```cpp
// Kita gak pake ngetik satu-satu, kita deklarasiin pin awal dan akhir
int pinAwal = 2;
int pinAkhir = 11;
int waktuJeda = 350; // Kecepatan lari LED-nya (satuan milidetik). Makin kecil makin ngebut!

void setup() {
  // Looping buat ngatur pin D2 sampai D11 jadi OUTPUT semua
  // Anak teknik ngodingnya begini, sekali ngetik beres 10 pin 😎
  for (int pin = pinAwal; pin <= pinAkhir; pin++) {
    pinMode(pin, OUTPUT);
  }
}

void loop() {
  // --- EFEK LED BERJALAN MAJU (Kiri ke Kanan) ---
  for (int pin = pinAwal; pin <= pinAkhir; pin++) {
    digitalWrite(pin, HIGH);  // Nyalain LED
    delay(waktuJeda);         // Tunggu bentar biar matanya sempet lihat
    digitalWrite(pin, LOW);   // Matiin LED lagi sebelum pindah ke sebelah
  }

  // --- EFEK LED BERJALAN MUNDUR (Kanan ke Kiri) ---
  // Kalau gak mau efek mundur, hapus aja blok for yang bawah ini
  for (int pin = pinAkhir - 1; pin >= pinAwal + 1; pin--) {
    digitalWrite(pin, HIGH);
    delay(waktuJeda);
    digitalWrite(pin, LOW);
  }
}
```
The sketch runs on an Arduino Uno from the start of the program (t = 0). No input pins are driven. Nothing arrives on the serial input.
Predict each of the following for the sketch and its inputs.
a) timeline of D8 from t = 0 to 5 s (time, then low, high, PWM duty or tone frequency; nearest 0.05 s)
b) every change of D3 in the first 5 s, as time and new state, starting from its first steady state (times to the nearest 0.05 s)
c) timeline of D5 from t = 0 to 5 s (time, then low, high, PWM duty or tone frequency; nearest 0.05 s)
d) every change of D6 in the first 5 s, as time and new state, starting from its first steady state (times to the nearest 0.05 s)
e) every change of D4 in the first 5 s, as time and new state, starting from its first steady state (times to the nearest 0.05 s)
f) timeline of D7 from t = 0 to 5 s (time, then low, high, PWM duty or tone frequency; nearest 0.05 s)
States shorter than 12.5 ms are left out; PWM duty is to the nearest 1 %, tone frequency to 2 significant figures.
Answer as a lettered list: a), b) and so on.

a) 0 s low; 2.1 s high; 2.45 s low; 4.2 s high; 4.55 s low
b) 0 s low; 0.35 s high; 0.7 s low
c) 0 s low; 1.05 s high; 1.4 s low
d) 0 s low; 1.4 s high; 1.75 s low; 4.9 s high
e) 0 s low; 0.7 s high; 1.05 s low
f) 0 s low; 1.75 s high; 2.1 s low; 4.55 s high; 4.9 s low
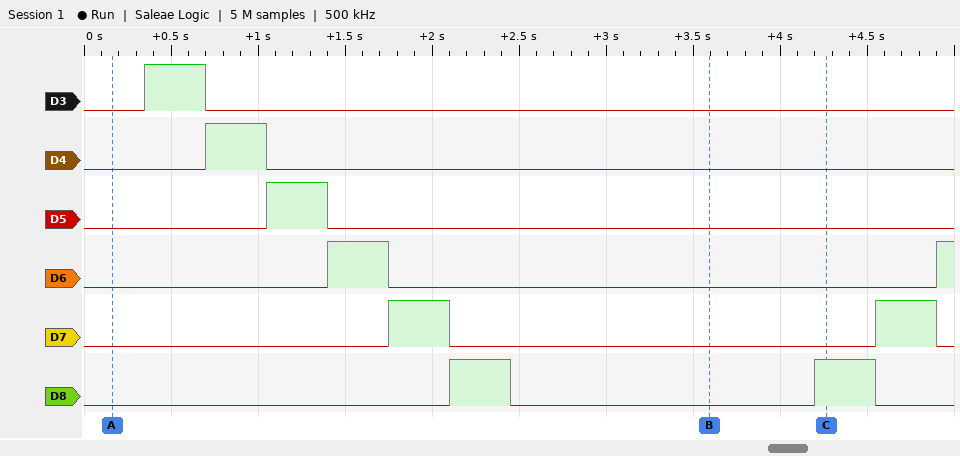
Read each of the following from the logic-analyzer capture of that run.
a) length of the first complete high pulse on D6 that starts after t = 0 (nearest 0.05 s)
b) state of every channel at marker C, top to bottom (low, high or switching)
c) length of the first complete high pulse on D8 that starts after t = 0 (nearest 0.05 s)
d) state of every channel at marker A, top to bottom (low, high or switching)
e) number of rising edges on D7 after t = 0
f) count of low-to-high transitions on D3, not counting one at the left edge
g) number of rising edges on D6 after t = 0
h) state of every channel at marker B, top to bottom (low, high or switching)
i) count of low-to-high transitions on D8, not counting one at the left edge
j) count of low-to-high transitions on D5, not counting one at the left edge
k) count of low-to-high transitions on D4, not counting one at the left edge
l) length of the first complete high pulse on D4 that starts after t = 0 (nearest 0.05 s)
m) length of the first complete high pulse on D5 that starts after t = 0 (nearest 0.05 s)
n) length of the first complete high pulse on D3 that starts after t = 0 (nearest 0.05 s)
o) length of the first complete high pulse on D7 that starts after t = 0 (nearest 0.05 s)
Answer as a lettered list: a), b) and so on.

a) 0.35 s
b) D3 low, D4 low, D5 low, D6 low, D7 low, D8 high
c) 0.35 s
d) D3 low, D4 low, D5 low, D6 low, D7 low, D8 low
e) 2
f) 1
g) 2
h) D3 low, D4 low, D5 low, D6 low, D7 low, D8 low
i) 2
j) 1
k) 1
l) 0.35 s
m) 0.35 s
n) 0.35 s
o) 0.35 s
